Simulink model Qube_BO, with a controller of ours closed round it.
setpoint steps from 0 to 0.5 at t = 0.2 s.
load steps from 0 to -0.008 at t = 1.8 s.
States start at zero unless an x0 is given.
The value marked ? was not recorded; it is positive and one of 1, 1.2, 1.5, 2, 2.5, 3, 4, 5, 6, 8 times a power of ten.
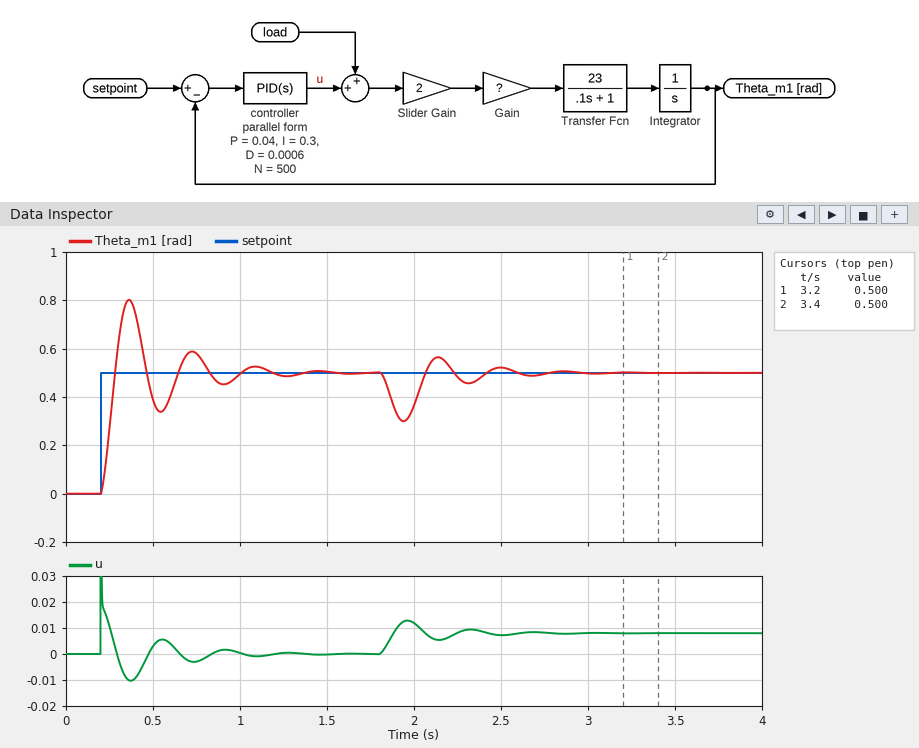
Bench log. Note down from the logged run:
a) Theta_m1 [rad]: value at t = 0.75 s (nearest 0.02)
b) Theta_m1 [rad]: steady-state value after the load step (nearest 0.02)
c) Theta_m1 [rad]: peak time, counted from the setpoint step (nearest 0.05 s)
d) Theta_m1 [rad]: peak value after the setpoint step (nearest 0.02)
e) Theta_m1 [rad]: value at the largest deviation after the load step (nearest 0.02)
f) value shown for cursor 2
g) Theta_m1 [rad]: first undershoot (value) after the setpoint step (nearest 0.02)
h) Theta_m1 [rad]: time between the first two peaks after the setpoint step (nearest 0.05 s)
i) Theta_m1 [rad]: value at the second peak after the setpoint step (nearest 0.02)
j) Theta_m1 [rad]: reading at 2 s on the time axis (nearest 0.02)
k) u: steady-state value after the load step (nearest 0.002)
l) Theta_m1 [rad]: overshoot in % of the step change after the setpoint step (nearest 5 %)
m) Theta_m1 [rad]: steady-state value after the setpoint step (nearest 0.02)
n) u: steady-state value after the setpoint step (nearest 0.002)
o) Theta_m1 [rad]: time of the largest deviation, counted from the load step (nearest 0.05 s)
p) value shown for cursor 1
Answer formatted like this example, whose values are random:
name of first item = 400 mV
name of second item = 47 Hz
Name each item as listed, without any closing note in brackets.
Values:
Theta_m1 [rad]: value at t = 0.75 s = 0.58
Theta_m1 [rad]: steady-state value after the load step = 0.50
Theta_m1 [rad]: peak time, counted from the setpoint step = 0.15 s
Theta_m1 [rad]: peak value after the setpoint step = 0.80
Theta_m1 [rad]: value at the largest deviation after the load step = 0.30
value shown for cursor 2 = 0.500
Theta_m1 [rad]: first undershoot (value) after the setpoint step = 0.34
Theta_m1 [rad]: time between the first two peaks after the setpoint step = 0.35 s
Theta_m1 [rad]: value at the second peak after the setpoint step = 0.58
Theta_m1 [rad]: reading at 2 s on the time axis = 0.36
u: steady-state value after the load step = 0.008
Theta_m1 [rad]: overshoot in % of the step change after the setpoint step = 60 %
Theta_m1 [rad]: steady-state value after the setpoint step = 0.50
u: steady-state value after the setpoint step = 0.000
Theta_m1 [rad]: time of the largest deviation, counted from the load step = 0.15 s
value shown for cursor 1 = 0.500
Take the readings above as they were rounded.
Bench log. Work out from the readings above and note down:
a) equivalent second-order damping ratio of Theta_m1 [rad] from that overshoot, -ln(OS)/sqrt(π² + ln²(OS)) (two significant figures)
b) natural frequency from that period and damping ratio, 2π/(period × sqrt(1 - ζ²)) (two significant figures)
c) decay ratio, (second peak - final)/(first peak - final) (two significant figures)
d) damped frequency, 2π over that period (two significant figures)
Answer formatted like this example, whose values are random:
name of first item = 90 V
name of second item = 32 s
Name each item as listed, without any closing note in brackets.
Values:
equivalent second-order damping ratio of Theta_m1 [rad] from that overshoot, -ln(OS)/sqrt(π² + ln²(OS)) = 0.16
natural frequency from that period and damping ratio, 2π/(period × sqrt(1 - ζ²)) = 18 rad/s
decay ratio, (second peak - final)/(first peak - final) = 0.27
damped frequency, 2π over that period = 18 rad/s
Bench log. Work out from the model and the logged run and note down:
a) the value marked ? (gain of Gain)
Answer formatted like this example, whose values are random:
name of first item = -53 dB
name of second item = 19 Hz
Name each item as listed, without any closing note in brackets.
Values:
the value marked ? = 20
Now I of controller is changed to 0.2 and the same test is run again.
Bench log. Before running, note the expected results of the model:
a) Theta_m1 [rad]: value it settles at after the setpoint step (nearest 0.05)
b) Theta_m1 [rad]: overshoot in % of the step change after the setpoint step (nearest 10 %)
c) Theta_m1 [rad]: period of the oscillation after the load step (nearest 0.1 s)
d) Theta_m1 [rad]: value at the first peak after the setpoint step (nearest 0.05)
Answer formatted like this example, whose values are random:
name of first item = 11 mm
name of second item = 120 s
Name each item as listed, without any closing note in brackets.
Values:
Theta_m1 [rad]: value it settles at after the setpoint step = 0.50
Theta_m1 [rad]: overshoot in % of the step change after the setpoint step = 50 %
Theta_m1 [rad]: period of the oscillation after the load step = 0.4 s
Theta_m1 [rad]: value at the first peak after the setpoint step = 0.75
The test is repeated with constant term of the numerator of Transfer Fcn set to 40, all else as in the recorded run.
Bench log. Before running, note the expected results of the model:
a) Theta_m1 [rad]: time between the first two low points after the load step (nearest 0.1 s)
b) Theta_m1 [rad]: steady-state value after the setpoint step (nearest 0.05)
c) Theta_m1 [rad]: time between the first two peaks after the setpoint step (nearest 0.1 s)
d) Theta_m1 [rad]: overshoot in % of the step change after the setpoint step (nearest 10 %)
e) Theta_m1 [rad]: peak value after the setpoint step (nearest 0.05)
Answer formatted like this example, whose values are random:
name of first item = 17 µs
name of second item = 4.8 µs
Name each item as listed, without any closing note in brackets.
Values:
Theta_m1 [rad]: time between the first two low points after the load step = 0.3 s
Theta_m1 [rad]: steady-state value after the setpoint step = 0.50
Theta_m1 [rad]: time between the first two peaks after the setpoint step = 0.3 s
Theta_m1 [rad]: overshoot in % of the step change after the setpoint step = 50 %
Theta_m1 [rad]: peak value after the setpoint step = 0.75
